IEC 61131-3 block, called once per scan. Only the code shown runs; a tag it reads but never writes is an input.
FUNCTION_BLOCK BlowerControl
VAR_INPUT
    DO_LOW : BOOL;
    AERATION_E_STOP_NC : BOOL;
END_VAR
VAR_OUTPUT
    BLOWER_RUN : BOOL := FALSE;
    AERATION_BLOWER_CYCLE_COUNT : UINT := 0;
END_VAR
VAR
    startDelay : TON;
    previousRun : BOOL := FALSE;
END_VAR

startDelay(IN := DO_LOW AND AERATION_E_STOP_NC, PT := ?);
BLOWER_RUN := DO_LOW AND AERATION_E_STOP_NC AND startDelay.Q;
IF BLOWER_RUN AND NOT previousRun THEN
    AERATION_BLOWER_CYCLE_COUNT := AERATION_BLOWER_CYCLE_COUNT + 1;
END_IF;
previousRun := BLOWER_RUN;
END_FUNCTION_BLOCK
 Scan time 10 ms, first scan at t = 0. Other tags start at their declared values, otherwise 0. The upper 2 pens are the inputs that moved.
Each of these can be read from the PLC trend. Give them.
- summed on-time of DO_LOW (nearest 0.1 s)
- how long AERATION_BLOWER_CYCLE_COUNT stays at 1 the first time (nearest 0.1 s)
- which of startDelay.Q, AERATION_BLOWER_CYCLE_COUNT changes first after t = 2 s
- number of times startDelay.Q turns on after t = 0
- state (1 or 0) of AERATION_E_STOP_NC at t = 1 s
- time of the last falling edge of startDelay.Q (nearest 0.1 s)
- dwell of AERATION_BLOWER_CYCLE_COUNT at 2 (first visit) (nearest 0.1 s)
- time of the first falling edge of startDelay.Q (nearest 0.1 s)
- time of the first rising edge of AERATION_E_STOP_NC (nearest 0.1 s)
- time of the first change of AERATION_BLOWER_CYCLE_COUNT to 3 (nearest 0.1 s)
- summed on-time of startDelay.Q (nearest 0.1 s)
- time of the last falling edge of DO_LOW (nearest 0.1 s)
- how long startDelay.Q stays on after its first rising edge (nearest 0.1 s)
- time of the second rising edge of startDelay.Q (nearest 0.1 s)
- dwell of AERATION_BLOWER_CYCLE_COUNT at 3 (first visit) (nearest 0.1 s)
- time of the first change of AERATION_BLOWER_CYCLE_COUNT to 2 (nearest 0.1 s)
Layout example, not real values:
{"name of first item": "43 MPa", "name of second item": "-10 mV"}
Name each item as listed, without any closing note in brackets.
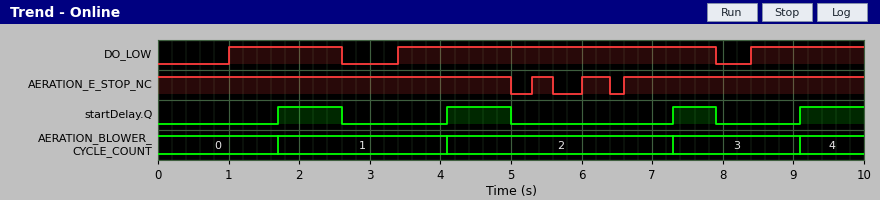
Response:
{"summed on-time of DO_LOW": "7.7 s", "how long AERATION_BLOWER_CYCLE_COUNT stays at 1 the first time": "2.4 s", "which of startDelay.Q, AERATION_BLOWER_CYCLE_COUNT changes first after t = 2 s": "startDelay.Q", "number of times startDelay.Q turns on after t = 0": "4", "state (1 or 0) of AERATION_E_STOP_NC at t = 1 s": "1", "time of the last falling edge of startDelay.Q": "7.9 s", "dwell of AERATION_BLOWER_CYCLE_COUNT at 2 (first visit)": "3.2 s", "time of the first falling edge of startDelay.Q": "2.6 s", "time of the first rising edge of AERATION_E_STOP_NC": "5.3 s", "time of the first change of AERATION_BLOWER_CYCLE_COUNT to 3": "7.3 s", "summed on-time of startDelay.Q": "3.3 s", "time of the last falling edge of DO_LOW": "7.9 s", "how long startDelay.Q stays on after its first rising edge": "0.9 s", "time of the second rising edge of startDelay.Q": "4.1 s", "dwell of AERATION_BLOWER_CYCLE_COUNT at 3 (first visit)": "1.8 s", "time of the first change of AERATION_BLOWER_CYCLE_COUNT to 2": "4.1 s"}
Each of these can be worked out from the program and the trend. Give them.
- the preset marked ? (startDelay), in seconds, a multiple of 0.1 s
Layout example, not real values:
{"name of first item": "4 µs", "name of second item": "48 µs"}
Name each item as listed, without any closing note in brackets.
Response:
{"the preset marked ? (startDelay), in seconds, a multiple of 0.1 s": "0.7 s"}
